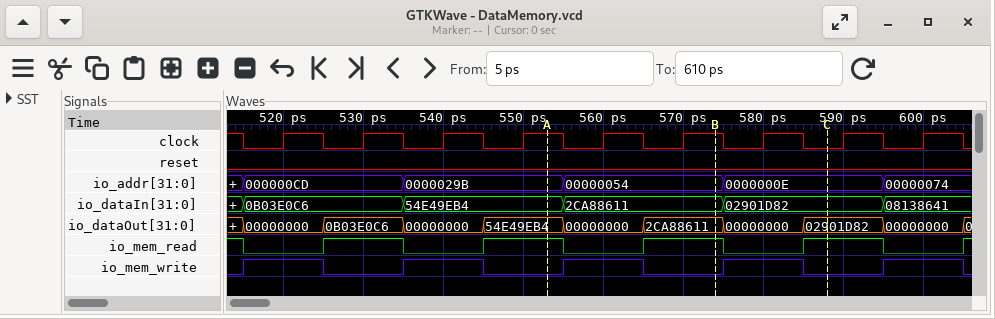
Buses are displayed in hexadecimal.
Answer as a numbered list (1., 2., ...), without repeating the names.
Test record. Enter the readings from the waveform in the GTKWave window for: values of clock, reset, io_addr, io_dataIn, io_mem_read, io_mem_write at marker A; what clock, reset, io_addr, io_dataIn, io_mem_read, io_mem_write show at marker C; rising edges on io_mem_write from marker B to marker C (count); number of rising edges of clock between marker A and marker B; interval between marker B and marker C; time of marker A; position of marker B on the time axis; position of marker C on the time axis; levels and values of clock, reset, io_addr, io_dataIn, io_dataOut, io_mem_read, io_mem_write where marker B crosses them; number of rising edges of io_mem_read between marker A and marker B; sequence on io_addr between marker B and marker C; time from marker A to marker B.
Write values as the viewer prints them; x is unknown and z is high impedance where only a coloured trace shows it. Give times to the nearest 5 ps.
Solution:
1. clock=1, reset=0, io_addr=0000029B, io_dataIn=54E49EB4, io_mem_read=1, io_mem_write=0
2. clock=0, reset=0, io_addr=0000000E, io_dataIn=02901D82, io_mem_read=1, io_mem_write=0
3. 1
4. 2
5. 15 ps
6. 555 ps
7. 575 ps
8. 590 ps
9. clock=1, reset=0, io_addr=00000054, io_dataIn=2CA88611, io_dataOut=2CA88611, io_mem_read=1, io_mem_write=0
10. 1
11. 00000054, 0000000E
12. 20 ps
